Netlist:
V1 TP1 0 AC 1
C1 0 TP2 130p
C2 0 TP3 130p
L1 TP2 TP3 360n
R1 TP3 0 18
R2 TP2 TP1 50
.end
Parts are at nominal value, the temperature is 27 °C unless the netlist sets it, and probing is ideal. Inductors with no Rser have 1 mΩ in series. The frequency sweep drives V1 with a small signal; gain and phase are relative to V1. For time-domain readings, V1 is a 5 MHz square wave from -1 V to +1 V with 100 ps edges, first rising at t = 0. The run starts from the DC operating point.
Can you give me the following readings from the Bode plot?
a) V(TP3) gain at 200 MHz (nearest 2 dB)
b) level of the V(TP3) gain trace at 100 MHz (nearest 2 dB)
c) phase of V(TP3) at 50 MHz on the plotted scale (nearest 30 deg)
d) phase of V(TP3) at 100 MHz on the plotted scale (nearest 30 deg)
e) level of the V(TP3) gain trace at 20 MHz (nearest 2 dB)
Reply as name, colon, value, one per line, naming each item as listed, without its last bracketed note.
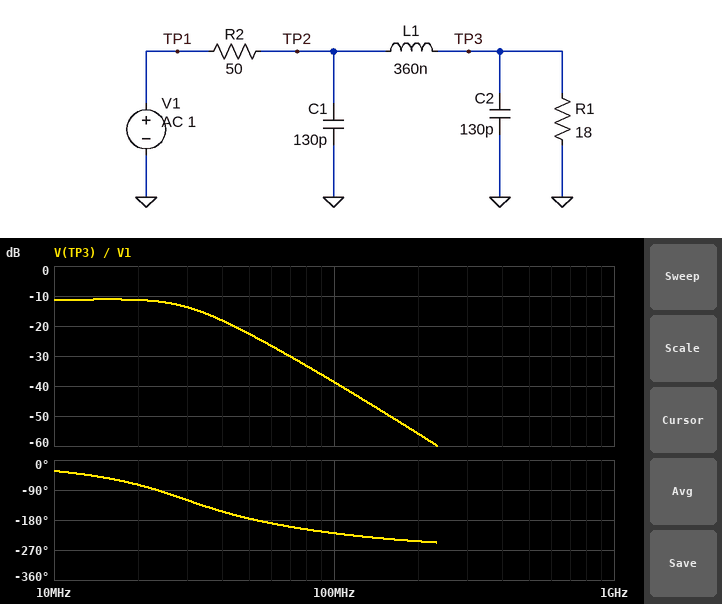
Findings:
V(TP3) gain at 200 MHz: -56 dB
level of the V(TP3) gain trace at 100 MHz: -38 dB
phase of V(TP3) at 50 MHz on the plotted scale: -180 deg
phase of V(TP3) at 100 MHz on the plotted scale: -210 deg
level of the V(TP3) gain trace at 20 MHz: -12 dB
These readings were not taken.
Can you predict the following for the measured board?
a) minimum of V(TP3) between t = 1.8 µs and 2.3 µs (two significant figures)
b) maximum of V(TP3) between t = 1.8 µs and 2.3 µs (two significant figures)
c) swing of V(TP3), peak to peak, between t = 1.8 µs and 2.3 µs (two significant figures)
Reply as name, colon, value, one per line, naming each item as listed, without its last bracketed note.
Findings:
minimum of V(TP3) between t = 1.8 µs and 2.3 µs: -320 mV
maximum of V(TP3) between t = 1.8 µs and 2.3 µs: 320 mV
swing of V(TP3), peak to peak, between t = 1.8 µs and 2.3 µs: 640 mV
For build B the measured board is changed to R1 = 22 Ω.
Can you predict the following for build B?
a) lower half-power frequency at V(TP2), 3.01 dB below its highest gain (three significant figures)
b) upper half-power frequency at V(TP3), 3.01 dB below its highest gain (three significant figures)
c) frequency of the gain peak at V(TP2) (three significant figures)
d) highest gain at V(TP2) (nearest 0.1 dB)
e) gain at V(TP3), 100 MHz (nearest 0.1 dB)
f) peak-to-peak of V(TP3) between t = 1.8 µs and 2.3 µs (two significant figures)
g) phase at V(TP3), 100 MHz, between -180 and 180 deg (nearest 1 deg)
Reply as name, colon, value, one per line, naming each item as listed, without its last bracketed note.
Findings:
lower half-power frequency at V(TP2), 3.01 dB below its highest gain: 15.8 MHz
upper half-power frequency at V(TP3), 3.01 dB below its highest gain: 31.8 MHz
frequency of the gain peak at V(TP2): 29.1 MHz
highest gain at V(TP2): -2.3 dB
gain at V(TP3), 100 MHz: -38.1 dB
peak-to-peak of V(TP3) between t = 1.8 µs and 2.3 µs: 740 mV
phase at V(TP3), 100 MHz, between -180 and 180 deg: 135 deg
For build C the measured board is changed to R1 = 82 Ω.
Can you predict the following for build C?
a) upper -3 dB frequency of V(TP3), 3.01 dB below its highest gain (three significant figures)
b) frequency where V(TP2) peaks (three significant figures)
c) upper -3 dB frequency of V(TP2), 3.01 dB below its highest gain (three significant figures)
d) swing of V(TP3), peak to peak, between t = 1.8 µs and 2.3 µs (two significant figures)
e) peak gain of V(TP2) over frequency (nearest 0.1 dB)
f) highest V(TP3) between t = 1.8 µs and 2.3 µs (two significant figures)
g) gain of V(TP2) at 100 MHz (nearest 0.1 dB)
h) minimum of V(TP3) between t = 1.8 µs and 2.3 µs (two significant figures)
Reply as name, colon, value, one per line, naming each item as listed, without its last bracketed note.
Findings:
upper -3 dB frequency of V(TP3), 3.01 dB below its highest gain: 35.6 MHz
frequency where V(TP2) peaks: 35.3 MHz
upper -3 dB frequency of V(TP2), 3.01 dB below its highest gain: 51.4 MHz
swing of V(TP3), peak to peak, between t = 1.8 µs and 2.3 µs: 1.5 V
peak gain of V(TP2) over frequency: -2.5 dB
highest V(TP3) between t = 1.8 µs and 2.3 µs: 750 mV
gain of V(TP2) at 100 MHz: -12.0 dB
minimum of V(TP3) between t = 1.8 µs and 2.3 µs: -750 mV
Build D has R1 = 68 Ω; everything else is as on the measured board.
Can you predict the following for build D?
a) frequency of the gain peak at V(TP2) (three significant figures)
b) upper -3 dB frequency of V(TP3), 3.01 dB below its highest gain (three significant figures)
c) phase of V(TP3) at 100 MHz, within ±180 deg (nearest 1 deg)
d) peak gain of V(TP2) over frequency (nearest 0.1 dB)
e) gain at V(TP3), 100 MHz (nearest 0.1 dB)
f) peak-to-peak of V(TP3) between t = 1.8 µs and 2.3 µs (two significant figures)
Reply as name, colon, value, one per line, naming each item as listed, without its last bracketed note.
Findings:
frequency of the gain peak at V(TP2): 35.2 MHz
upper -3 dB frequency of V(TP3), 3.01 dB below its highest gain: 35.6 MHz
phase of V(TP3) at 100 MHz, within ±180 deg: 115 deg
peak gain of V(TP2) over frequency: -2.6 dB
gain at V(TP3), 100 MHz: -37.0 dB
peak-to-peak of V(TP3) between t = 1.8 µs and 2.3 µs: 1.4 V
